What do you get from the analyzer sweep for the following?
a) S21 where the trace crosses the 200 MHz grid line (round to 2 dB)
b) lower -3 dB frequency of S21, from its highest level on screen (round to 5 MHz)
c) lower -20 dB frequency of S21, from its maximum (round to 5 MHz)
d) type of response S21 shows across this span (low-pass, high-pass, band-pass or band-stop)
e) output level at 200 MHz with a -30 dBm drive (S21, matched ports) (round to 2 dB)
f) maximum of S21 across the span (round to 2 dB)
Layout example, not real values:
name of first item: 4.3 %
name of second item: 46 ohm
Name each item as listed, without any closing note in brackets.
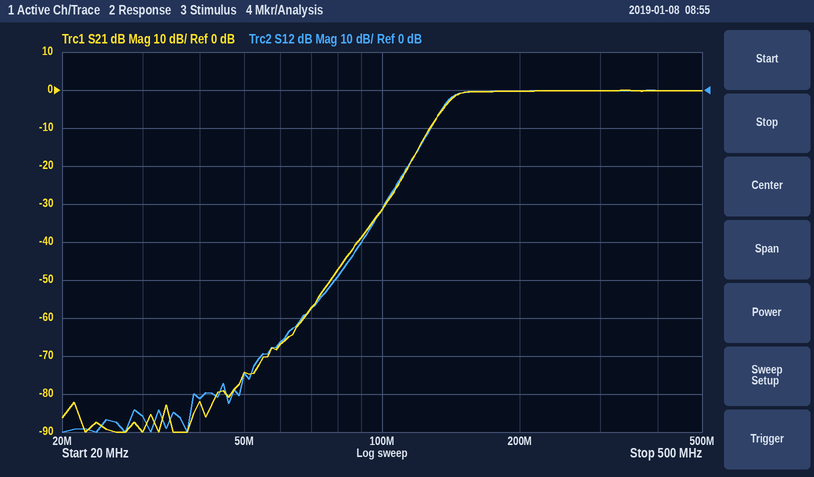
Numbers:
S21 where the trace crosses the 200 MHz grid line: 0 dB
lower -3 dB frequency of S21, from its highest level on screen: 140 MHz
lower -20 dB frequency of S21, from its maximum: 115 MHz
type of response S21 shows across this span: high-pass
output level at 200 MHz with a -30 dBm drive (S21, matched ports): -30 dBm
maximum of S21 across the span: 0 dB
